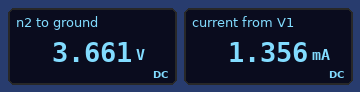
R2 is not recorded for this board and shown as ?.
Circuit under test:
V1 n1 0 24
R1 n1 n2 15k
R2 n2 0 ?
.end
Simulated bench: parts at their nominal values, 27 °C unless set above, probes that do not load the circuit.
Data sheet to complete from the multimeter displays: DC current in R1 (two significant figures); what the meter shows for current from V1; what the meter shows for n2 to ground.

1.4 mA
1.356 mA
3.661 V
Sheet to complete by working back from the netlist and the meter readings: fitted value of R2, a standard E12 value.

2.7 kΩ
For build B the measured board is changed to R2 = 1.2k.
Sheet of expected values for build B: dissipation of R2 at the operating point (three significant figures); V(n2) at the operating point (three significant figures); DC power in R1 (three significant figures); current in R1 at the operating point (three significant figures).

2.63 mW
1.78 V
32.9 mW
1.48 mA
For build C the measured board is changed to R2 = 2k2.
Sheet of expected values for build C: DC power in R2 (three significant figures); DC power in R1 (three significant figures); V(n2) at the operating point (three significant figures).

4.28 mW
29.2 mW
3.07 V
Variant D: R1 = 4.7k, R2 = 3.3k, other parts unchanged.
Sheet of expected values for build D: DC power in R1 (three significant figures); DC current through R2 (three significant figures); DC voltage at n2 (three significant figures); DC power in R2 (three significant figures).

42.3 mW
3.00 mA
9.90 V
29.7 mW
